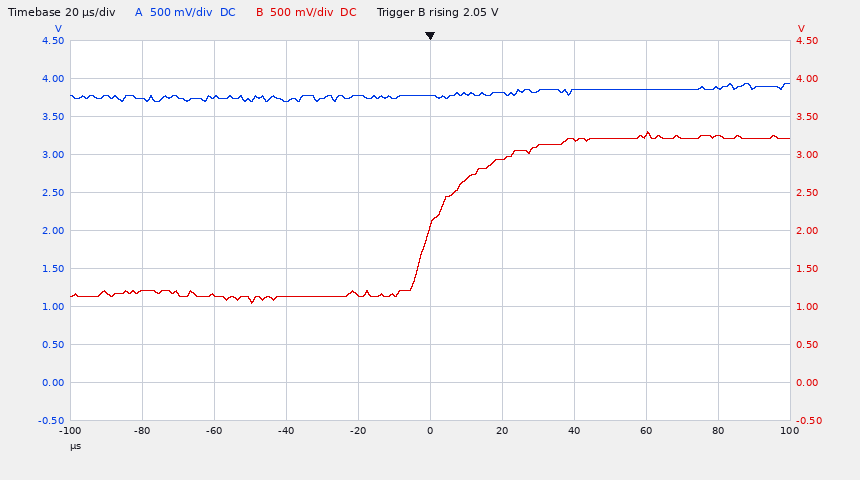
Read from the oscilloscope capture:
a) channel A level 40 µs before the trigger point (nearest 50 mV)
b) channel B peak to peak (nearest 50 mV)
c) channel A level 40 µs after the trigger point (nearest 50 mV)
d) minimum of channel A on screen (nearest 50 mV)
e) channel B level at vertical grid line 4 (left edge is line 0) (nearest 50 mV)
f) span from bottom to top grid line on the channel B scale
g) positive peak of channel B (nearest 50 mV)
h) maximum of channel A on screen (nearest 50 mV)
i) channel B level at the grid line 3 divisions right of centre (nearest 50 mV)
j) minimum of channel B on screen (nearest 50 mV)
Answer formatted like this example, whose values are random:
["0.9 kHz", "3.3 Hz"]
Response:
["3.70 V", "2.25 V", "3.85 V", "3.70 V", "1.15 V", "5 V", "3.30 V", "3.95 V", "3.25 V", "1.05 V"]
